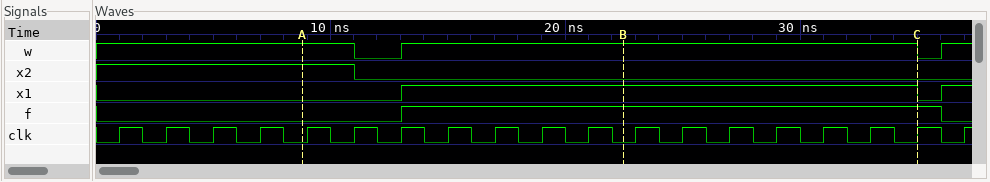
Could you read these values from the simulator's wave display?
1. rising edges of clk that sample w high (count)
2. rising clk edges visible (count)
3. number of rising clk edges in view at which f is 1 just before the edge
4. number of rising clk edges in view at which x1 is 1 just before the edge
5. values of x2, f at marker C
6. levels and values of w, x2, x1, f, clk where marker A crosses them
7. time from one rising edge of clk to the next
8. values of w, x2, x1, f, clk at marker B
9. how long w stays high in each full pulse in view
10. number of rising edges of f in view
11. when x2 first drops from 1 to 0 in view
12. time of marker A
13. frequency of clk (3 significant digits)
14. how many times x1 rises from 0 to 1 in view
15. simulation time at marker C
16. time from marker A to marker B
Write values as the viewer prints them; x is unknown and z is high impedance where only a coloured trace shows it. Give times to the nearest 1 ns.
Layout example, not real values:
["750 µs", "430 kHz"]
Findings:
["18", "19", "11", "12", "x2=0, f=1", "w=1, x2=1, x1=0, f=0, clk=0", "2 ns", "w=1, x2=0, x1=1, f=1, clk=0", "22 ns", "1", "11 ns", "9 ns", "500 MHz", "2", "35 ns", "14 ns"]
